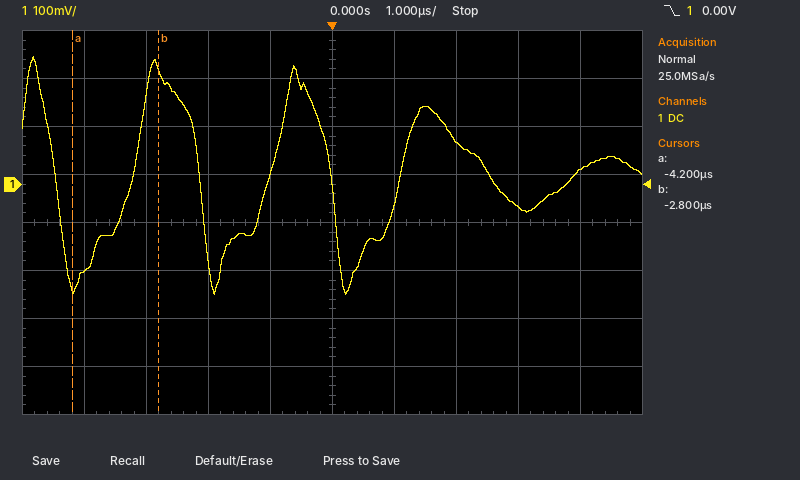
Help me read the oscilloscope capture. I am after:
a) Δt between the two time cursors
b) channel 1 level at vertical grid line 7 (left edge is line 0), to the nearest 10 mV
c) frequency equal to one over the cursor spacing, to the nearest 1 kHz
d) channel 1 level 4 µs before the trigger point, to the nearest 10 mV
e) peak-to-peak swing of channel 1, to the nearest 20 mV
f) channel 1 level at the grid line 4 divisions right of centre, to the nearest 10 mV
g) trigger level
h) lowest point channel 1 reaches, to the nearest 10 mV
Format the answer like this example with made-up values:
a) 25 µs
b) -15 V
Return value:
a) 1.4 µs
b) 90 mV
c) 714 kHz
d) -180 mV
e) 500 mV
f) 30 mV
g) 0.00 V
h) -230 mV
